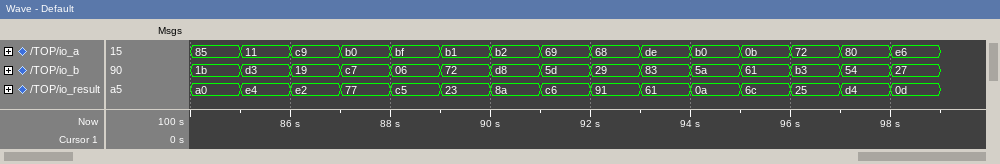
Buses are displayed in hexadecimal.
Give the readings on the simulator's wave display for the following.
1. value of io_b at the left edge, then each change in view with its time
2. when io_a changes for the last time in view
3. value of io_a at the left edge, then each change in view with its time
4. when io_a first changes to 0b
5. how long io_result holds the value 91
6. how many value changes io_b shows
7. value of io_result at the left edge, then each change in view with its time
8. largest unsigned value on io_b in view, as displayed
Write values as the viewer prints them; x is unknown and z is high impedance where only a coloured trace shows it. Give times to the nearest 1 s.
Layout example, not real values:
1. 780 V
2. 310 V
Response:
1. 1b, d3 at 85 s, 19 at 86 s, c7 at 87 s, 06 at 88 s, 72 at 89 s, d8 at 90 s, 5d at 91 s, 29 at 92 s, 83 at 93 s, 5a at 94 s, 61 at 95 s, b3 at 96 s, 54 at 97 s, 27 at 98 s
2. 98 s
3. 85, 11 at 85 s, c9 at 86 s, b0 at 87 s, bf at 88 s, b1 at 89 s, b2 at 90 s, 69 at 91 s, 68 at 92 s, de at 93 s, b0 at 94 s, 0b at 95 s, 72 at 96 s, 80 at 97 s, e6 at 98 s
4. 95 s
5. 1 s
6. 14
7. a0, e4 at 85 s, e2 at 86 s, 77 at 87 s, c5 at 88 s, 23 at 89 s, 8a at 90 s, c6 at 91 s, 91 at 92 s, 61 at 93 s, 0a at 94 s, 6c at 95 s, 25 at 96 s, d4 at 97 s, 0d at 98 s
8. d8
